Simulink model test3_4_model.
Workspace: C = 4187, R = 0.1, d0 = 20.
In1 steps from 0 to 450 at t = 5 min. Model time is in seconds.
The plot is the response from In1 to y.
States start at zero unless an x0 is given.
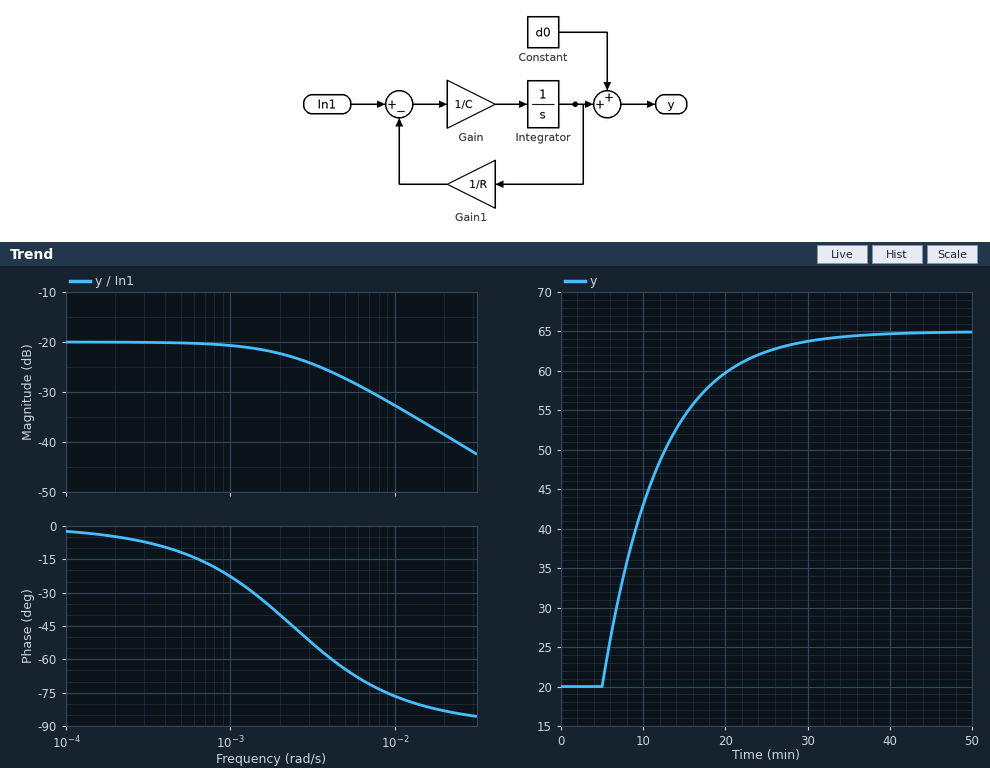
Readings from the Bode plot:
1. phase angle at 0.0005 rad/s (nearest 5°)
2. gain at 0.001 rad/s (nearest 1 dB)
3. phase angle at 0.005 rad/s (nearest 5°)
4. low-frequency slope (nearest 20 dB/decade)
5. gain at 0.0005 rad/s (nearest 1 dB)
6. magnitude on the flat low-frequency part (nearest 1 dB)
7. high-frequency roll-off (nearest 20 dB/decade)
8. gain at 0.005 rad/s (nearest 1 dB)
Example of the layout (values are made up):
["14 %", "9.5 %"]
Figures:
["-10°", "-21 dB", "-65°", "0 dB/decade", "-20 dB", "-20 dB", "-20 dB/decade", "-27 dB"]
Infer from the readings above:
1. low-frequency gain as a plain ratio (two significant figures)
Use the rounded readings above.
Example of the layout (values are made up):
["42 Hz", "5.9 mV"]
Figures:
["0.10"]
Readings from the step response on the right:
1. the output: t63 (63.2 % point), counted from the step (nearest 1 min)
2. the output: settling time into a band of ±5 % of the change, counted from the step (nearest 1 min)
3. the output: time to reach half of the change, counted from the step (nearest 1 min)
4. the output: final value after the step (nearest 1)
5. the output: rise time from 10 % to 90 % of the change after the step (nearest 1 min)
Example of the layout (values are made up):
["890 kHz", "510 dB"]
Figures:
["7 min", "21 min", "5 min", "65", "15 min"]
